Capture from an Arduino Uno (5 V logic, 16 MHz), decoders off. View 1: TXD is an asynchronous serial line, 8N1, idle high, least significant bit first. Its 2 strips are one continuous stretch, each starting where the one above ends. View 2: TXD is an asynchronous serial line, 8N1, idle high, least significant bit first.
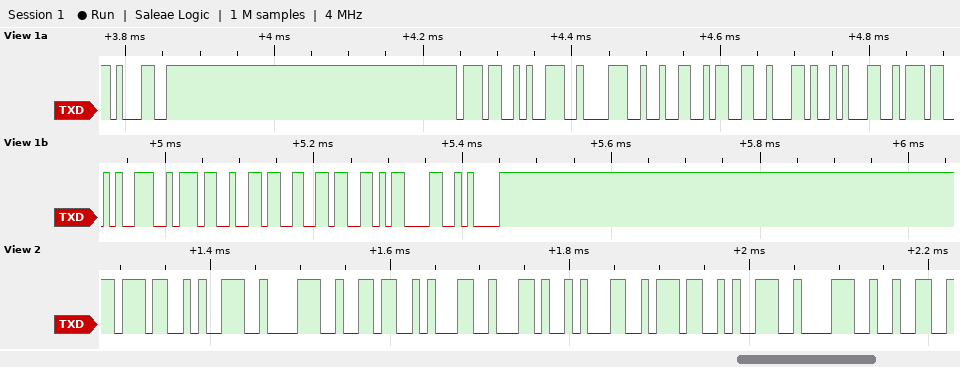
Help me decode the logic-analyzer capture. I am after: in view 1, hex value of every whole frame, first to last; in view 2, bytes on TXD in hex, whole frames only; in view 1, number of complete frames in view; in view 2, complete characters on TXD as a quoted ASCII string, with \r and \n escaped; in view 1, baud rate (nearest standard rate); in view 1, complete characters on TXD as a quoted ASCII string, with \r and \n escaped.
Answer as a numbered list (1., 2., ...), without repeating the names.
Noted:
1. 31 37 39 38 32 33 2C 31 37 39 37 36 36 0D 0A
2. 37 39 38 36 31 2C 31 37 39 38 32
3. 15
4. "79861,17982"
5. 115200 baud
6. "179823,179766\r\n"
